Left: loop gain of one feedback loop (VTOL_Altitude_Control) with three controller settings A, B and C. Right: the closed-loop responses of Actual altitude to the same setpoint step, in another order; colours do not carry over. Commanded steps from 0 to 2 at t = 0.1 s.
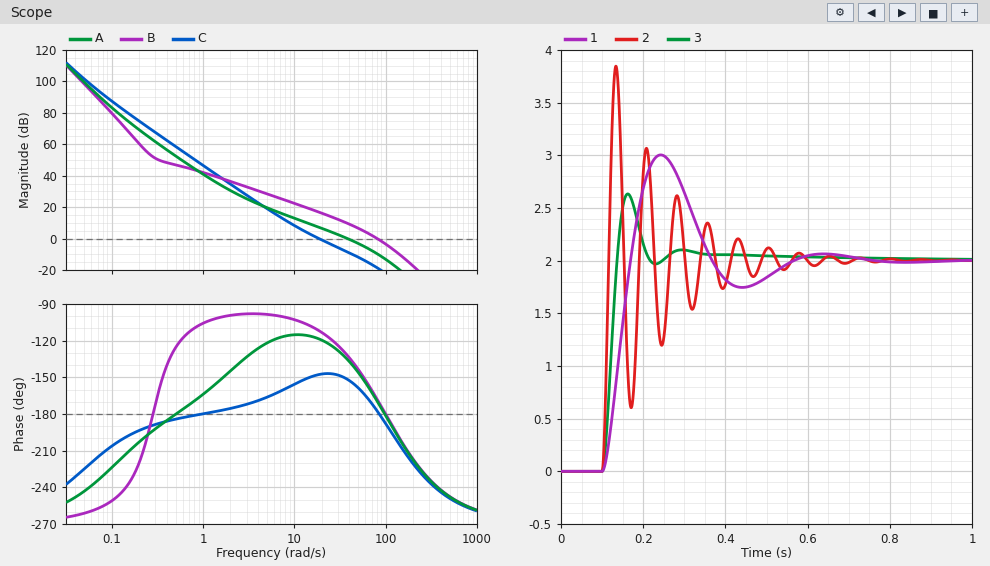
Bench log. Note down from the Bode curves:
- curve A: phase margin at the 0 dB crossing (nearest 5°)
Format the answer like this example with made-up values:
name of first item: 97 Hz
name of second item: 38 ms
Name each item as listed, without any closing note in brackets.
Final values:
curve A: phase margin at the 0 dB crossing: 45°
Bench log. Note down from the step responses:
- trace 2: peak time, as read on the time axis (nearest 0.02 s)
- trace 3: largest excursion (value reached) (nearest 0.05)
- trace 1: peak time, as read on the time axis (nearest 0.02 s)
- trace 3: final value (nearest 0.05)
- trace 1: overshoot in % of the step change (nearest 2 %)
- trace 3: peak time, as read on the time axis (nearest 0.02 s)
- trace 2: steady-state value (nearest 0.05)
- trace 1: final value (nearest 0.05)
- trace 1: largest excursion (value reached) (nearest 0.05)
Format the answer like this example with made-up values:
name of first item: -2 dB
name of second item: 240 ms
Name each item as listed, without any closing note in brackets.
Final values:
trace 2: peak time, as read on the time axis: 0.14 s
trace 3: largest excursion (value reached): 2.65
trace 1: peak time, as read on the time axis: 0.24 s
trace 3: final value: 2.00
trace 1: overshoot in % of the step change: 50 %
trace 3: peak time, as read on the time axis: 0.16 s
trace 2: steady-state value: 2.00
trace 1: final value: 2.00
trace 1: largest excursion (value reached): 3.00
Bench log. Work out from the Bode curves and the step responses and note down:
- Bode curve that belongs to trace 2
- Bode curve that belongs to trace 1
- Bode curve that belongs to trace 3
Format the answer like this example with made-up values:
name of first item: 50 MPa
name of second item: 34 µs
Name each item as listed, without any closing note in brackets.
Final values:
Bode curve that belongs to trace 2: B
Bode curve that belongs to trace 1: C
Bode curve that belongs to trace 3: A
